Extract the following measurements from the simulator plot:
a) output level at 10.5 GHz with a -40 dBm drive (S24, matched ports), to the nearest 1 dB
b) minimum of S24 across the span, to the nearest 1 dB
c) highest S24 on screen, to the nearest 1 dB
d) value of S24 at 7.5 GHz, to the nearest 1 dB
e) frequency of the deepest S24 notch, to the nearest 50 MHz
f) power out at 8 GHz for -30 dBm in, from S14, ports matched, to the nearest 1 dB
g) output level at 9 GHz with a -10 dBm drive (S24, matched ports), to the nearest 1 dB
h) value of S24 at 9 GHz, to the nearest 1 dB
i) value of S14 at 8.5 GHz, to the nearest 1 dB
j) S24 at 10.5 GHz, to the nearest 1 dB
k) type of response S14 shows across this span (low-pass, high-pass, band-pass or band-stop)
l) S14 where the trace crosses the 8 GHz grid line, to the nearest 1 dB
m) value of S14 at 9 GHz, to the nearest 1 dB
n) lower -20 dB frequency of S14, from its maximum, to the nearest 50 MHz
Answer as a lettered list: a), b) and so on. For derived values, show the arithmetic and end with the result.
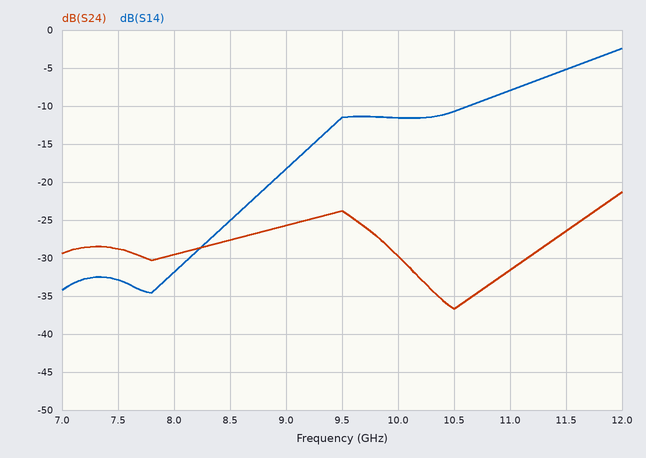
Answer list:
a) -40 dBm + (-37 dB) = -77 dBm
b) -37 dB
c) -21 dB
d) -29 dB
e) 10.50 GHz
f) -30 dBm + (-32 dB) = -62 dBm
g) -10 dBm + (-26 dB) = -36 dBm
h) -26 dB
i) -25 dB
j) -37 dB
k) high-pass
l) -32 dB
m) -18 dB
n) 8.70 GHz
